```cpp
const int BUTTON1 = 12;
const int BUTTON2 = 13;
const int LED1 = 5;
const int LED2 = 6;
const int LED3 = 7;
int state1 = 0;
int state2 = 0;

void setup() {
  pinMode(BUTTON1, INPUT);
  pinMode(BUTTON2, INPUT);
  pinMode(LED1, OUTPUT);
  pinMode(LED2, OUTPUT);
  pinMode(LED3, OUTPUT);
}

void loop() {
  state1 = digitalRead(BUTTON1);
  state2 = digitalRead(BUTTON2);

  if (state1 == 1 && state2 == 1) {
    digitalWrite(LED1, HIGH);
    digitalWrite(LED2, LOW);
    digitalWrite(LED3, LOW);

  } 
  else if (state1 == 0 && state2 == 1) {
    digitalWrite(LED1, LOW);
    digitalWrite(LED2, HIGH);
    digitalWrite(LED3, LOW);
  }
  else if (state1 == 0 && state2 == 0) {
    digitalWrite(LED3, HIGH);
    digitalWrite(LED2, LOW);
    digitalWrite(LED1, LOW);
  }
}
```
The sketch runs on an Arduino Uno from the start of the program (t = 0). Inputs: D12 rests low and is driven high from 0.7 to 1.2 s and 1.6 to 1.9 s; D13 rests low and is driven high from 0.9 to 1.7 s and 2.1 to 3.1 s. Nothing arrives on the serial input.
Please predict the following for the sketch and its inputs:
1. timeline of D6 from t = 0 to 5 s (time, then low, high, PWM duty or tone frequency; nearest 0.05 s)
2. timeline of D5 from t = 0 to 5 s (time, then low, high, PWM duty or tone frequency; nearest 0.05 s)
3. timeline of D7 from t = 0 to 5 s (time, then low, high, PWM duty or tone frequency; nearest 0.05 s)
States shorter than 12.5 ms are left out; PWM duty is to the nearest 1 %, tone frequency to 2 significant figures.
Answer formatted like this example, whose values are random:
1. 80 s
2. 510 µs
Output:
1. 0 s low; 1.2 s high; 1.6 s low; 2.1 s high; 3.1 s low
2. 0 s low; 0.9 s high; 1.2 s low; 1.6 s high; 1.9 s low
3. 0 s high; 0.9 s low; 1.9 s high; 2.1 s low; 3.1 s high
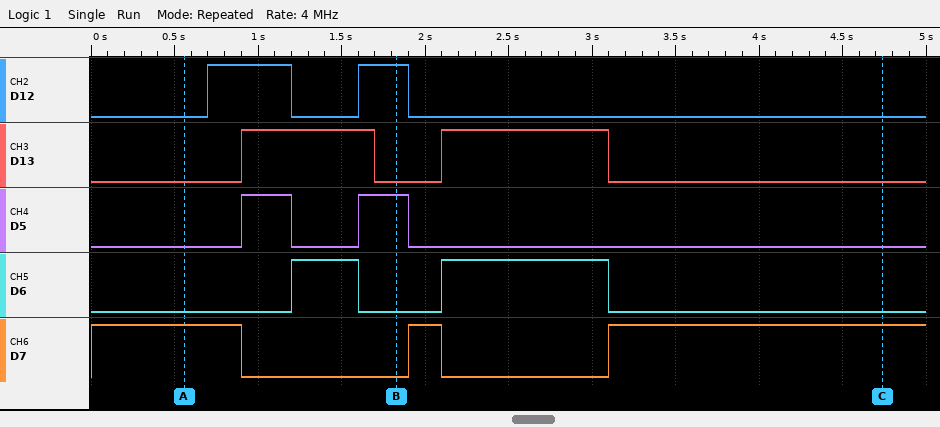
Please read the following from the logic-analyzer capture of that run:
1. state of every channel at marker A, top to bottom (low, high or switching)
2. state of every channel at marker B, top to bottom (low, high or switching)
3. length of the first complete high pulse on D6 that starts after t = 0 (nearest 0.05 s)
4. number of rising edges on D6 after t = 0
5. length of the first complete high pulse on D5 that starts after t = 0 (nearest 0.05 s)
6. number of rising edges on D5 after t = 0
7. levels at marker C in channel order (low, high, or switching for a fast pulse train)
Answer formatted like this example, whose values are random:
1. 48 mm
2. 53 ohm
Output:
1. D12 low, D13 low, D5 low, D6 low, D7 high
2. D12 high, D13 low, D5 high, D6 low, D7 low
3. 0.40 s
4. 2
5. 0.30 s
6. 2
7. D12 low, D13 low, D5 low, D6 low, D7 high
